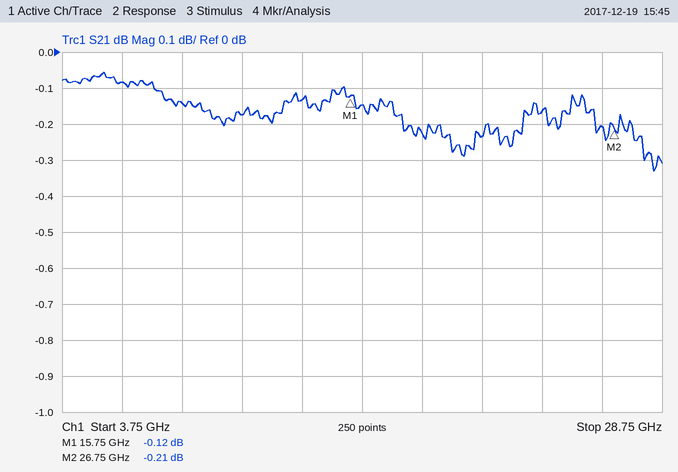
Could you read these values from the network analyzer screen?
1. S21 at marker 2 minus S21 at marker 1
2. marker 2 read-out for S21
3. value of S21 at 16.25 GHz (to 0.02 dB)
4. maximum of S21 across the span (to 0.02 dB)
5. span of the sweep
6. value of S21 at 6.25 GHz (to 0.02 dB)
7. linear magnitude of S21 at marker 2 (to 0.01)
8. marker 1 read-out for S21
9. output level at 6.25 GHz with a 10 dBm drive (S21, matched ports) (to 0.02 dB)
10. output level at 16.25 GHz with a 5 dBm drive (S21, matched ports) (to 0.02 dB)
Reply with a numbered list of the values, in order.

1. -0.09 dB
2. -0.21 dB
3. -0.14 dB
4. -0.06 dB
5. 25 GHz
6. -0.08 dB
7. 0.98
8. -0.12 dB
9. 9.92 dBm
10. 4.86 dBm
